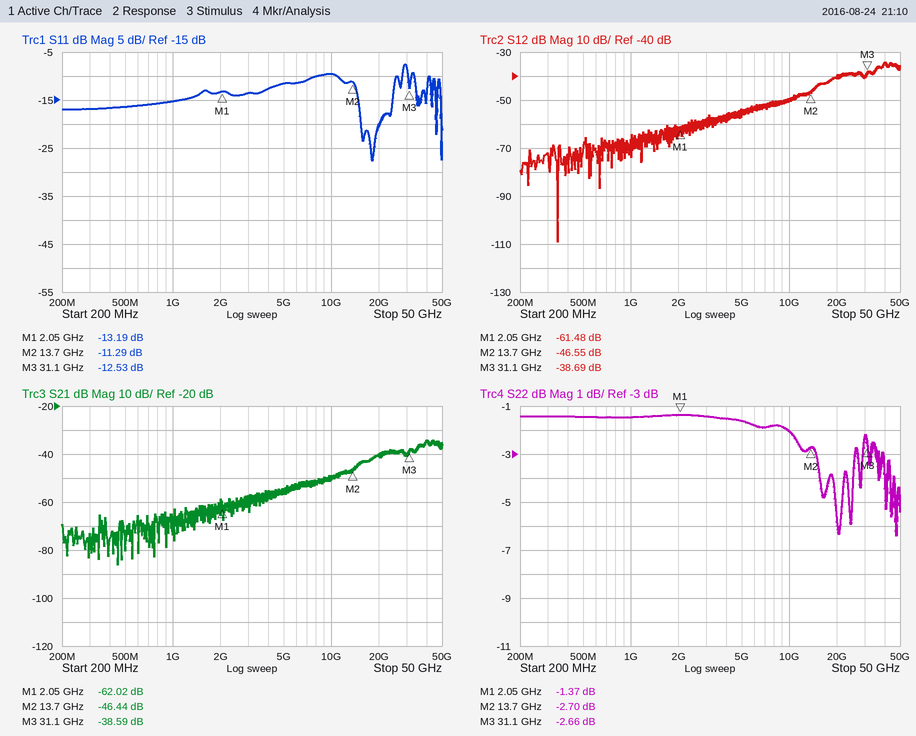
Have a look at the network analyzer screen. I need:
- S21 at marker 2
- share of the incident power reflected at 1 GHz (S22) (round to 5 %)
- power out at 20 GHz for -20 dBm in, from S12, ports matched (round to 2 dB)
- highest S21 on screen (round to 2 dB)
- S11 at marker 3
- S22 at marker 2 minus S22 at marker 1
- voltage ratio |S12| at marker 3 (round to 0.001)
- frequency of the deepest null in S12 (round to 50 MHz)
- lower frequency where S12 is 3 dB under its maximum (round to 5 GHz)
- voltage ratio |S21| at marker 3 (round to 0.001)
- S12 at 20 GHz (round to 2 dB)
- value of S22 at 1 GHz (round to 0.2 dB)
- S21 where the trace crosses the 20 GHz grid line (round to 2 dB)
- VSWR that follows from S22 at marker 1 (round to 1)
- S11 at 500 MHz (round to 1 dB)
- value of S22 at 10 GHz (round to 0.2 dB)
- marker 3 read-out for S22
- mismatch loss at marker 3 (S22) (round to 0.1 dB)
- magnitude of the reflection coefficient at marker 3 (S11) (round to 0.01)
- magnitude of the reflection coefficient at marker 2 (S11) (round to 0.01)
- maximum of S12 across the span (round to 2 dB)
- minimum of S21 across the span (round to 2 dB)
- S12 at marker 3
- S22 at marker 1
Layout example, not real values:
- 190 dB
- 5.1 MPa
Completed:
- -46.44 dB
- 70 %
- -60 dBm
- -34 dB
- -12.53 dB
- -1.33 dB
- 0.012
- 350 MHz
- 35 GHz
- 0.012
- -40 dB
- -1.4 dB
- -40 dB
- 13
- -16 dB
- -2.0 dB
- -2.66 dB
- 3.4 dB
- 0.24
- 0.27
- -34 dB
- -86 dB
- -38.69 dB
- -1.37 dB
